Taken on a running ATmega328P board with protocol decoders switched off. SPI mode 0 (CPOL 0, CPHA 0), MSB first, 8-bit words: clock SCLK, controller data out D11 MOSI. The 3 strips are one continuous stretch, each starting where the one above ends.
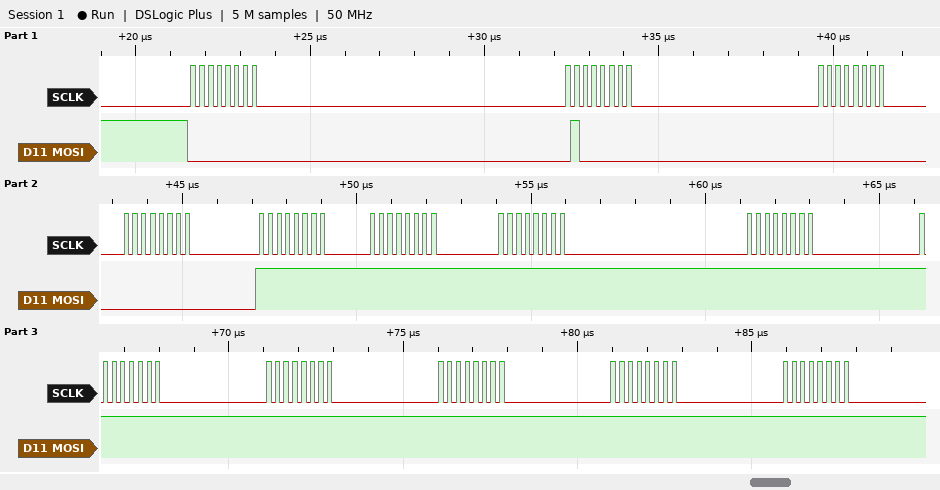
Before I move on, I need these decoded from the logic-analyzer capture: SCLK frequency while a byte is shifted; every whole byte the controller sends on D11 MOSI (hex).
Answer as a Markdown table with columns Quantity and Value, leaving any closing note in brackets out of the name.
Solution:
| Quantity | Value |
|---|---|
| SCLK frequency while a byte is shifted | 4 MHz |
| every whole byte the controller sends on D11 MOSI | 0x00 0x40 0x00 0x00 0xFF 0xFF 0xFF 0xFF 0xFF 0xFF 0xFF 0xFF 0xFF |
